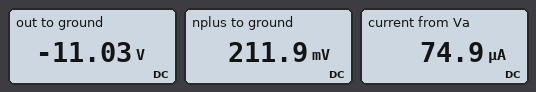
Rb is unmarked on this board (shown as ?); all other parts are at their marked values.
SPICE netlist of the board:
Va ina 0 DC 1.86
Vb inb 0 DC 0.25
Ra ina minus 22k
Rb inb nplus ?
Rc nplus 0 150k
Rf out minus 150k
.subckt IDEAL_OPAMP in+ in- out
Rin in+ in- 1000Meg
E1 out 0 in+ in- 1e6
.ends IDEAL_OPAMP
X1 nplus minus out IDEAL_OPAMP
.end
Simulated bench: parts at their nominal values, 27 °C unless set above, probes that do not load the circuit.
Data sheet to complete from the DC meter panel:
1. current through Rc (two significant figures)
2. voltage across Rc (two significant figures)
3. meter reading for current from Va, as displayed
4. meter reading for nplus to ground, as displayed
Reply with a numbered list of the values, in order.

1. 1.4 µA
2. 210 mV
3. 74.9 µA
4. 211.9 mV
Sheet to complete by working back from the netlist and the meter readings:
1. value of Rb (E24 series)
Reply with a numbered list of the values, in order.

1. 27 kΩ
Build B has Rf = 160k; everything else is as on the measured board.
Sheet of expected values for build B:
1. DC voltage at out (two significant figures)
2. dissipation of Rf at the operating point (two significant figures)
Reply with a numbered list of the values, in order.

1. -12 V
2. 900 µW
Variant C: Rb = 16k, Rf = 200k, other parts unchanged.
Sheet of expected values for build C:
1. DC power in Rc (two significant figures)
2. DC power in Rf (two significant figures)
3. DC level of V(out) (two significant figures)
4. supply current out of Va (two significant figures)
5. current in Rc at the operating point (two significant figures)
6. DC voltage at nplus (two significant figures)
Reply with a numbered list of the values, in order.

1. 340 nW
2. 1.1 mW
3. -15 V
4. 74 µA
5. 1.5 µA
6. 230 mV
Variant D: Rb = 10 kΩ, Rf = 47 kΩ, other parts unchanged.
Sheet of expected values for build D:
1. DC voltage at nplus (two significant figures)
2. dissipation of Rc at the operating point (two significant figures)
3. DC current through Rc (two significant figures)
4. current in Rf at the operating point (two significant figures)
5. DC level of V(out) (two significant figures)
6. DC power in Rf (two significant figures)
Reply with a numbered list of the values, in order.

1. 230 mV
2. 370 nW
3. 1.6 µA
4. 74 µA
5. -3.2 V
6. 260 µW
